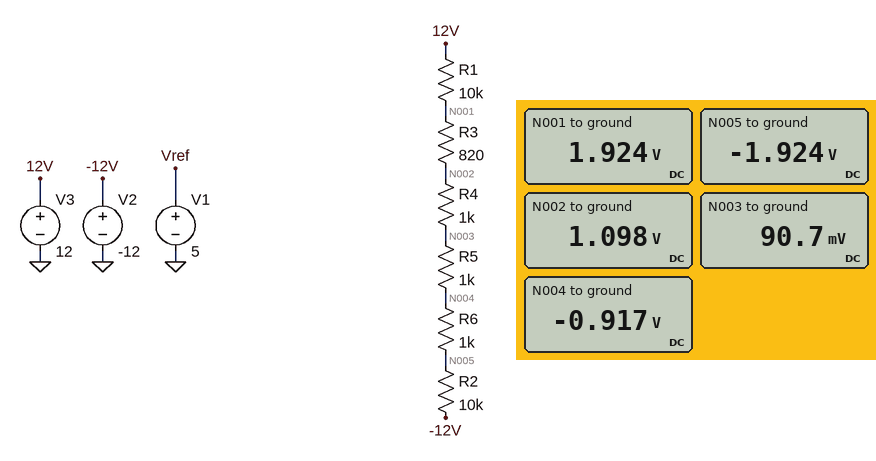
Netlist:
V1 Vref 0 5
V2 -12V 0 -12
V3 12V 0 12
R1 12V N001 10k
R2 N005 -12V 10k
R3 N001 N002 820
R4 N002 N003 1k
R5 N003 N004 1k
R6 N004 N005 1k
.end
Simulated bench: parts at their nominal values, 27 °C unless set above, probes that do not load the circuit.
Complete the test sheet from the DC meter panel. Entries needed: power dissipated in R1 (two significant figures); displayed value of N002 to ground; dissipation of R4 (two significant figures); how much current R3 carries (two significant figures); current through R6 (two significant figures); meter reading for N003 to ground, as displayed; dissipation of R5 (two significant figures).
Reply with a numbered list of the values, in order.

1. 10 mW
2. 1.098 V
3. 1.0 mW
4. 1.0 mA
5. 1.0 mA
6. 90.7 mV
7. 1.0 mW
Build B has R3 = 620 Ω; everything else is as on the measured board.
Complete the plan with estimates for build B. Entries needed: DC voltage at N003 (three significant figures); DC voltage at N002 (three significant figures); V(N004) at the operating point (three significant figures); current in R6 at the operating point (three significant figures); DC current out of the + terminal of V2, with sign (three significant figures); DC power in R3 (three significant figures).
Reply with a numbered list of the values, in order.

1. 193 mV
2. 1.21 V
3. -823 mV
4. 1.02 mA
5. -1.02 mA
6. 640 µW
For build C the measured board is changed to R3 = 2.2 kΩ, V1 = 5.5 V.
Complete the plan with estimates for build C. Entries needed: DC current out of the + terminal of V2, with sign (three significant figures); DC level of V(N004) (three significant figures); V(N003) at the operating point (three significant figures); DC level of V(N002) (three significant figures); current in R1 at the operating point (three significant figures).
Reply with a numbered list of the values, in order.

1. -952 µA
2. -1.52 V
3. -571 mV
4. 381 mV
5. 952 µA
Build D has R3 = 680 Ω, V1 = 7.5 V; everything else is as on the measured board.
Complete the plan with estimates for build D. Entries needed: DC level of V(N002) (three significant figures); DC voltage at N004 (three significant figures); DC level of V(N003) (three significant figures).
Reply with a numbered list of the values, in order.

1. 1.18 V
2. -851 mV
3. 162 mV
